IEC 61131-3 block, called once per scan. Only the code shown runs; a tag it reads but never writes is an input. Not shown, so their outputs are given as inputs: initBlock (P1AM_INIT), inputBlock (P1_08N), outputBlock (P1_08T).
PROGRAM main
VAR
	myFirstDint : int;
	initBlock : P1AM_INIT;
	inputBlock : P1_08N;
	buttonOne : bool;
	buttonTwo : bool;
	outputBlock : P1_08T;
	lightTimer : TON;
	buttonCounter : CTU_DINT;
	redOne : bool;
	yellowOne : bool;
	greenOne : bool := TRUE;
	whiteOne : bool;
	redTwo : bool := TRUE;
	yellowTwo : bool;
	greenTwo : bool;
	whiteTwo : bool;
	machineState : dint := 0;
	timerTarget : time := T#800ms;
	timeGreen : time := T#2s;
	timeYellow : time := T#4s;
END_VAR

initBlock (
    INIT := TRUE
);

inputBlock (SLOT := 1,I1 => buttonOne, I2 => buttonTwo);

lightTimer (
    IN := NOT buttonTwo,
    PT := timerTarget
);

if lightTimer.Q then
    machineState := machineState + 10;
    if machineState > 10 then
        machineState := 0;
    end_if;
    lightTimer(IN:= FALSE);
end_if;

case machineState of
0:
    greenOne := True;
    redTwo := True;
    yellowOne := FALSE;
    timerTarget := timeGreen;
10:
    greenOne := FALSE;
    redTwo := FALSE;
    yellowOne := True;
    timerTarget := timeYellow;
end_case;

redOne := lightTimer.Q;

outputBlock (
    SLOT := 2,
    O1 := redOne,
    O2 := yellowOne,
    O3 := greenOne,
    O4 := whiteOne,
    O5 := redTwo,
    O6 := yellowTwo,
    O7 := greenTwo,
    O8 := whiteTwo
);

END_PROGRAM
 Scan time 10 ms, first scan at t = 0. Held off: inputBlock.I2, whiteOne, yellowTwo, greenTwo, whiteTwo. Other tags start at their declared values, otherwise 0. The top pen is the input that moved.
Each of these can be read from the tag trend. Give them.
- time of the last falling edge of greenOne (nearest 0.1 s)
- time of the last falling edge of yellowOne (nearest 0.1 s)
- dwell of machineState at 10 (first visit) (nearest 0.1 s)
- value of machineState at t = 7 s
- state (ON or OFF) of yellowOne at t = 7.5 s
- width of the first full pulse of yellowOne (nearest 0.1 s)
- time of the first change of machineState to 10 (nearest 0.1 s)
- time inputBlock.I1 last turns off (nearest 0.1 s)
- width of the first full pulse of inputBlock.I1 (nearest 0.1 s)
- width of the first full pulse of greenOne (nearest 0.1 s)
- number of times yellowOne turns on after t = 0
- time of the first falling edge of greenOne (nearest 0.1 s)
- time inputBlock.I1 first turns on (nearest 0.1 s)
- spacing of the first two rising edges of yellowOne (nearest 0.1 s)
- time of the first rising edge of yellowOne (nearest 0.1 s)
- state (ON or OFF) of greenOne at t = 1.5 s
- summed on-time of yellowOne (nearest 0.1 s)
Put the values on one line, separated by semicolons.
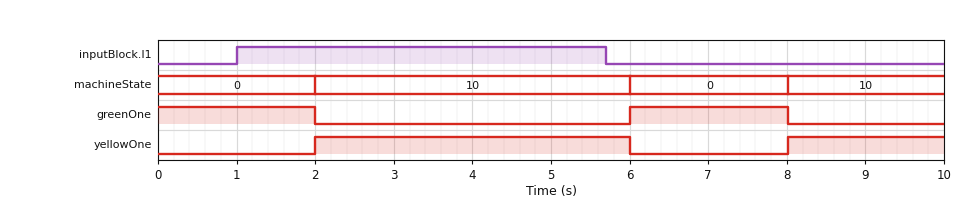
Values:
8.0 s; 6.0 s; 4.0 s; 0; OFF; 4.0 s; 2.0 s; 5.7 s; 4.7 s; 2.0 s; 2; 2.0 s; 1.0 s; 6.0 s; 2.0 s; ON; 6.0 s
